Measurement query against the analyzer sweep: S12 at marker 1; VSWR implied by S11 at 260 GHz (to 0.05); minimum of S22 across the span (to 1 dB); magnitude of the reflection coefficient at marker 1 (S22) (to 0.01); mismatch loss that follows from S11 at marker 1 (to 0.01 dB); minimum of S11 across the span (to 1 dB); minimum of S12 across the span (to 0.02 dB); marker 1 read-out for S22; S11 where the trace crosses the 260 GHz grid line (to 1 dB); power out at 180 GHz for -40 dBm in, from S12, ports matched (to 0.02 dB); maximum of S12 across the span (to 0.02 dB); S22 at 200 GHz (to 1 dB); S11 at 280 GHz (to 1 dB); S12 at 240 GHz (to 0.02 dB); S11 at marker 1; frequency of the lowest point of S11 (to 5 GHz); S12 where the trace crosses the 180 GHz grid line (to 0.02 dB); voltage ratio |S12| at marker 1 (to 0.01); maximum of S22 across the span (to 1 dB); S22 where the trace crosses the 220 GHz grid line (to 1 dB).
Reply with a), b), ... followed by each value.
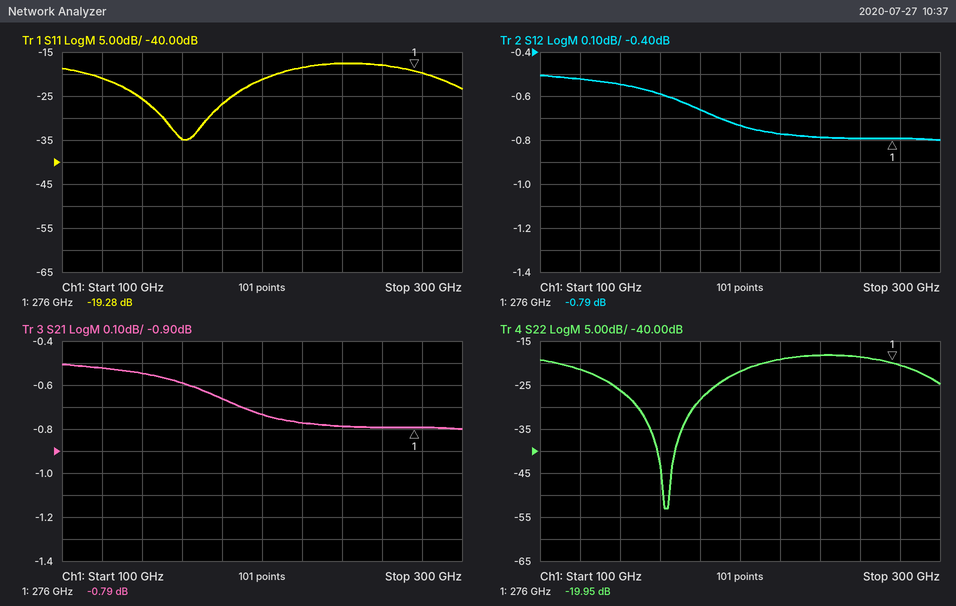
a) -0.79 dB
b) 1.30
c) -53 dB
d) 0.10
e) 0.05 dB
f) -35 dB
g) -0.80 dB
h) -19.95 dB
i) -18 dB
j) -40.66 dBm
k) -0.50 dB
l) -22 dB
m) -20 dB
n) -0.78 dB
o) -19.28 dB
p) 160 GHz
q) -0.66 dB
r) 0.91
s) -18 dB
t) -19 dB
